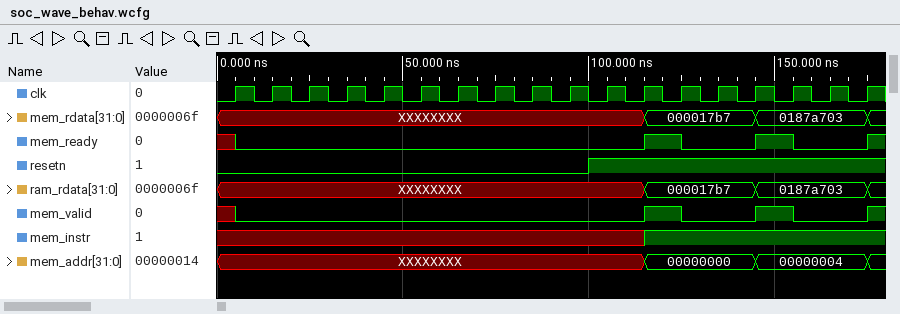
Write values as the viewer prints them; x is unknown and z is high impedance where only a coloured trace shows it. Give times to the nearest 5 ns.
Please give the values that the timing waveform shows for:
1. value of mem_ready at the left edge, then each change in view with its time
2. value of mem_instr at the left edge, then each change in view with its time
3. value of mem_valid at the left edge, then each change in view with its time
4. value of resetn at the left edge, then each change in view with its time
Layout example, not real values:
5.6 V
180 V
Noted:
x, 0 at 5 ns, 1 at 115 ns, 0 at 125 ns, 1 at 145 ns, 0 at 155 ns, 1 at 175 ns
x, 1 at 115 ns
x, 0 at 5 ns, 1 at 115 ns, 0 at 125 ns, 1 at 145 ns, 0 at 155 ns, 1 at 175 ns
0, 1 at 100 ns
